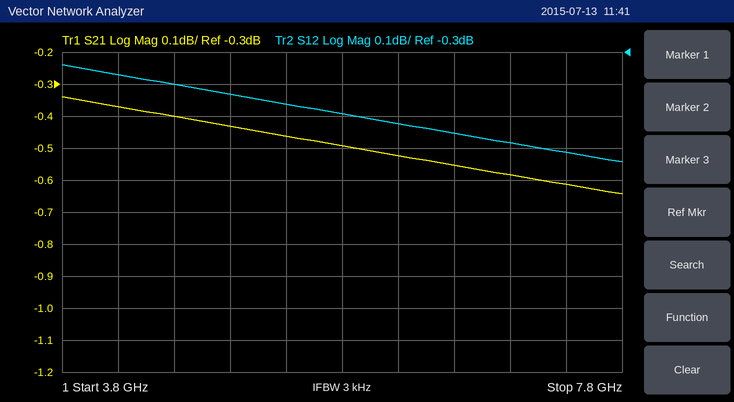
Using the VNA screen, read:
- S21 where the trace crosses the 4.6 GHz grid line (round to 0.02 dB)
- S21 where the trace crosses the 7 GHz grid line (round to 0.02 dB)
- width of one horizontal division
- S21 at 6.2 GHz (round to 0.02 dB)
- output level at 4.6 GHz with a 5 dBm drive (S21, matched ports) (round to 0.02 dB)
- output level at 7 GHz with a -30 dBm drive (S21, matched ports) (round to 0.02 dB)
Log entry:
-0.40 dB
-0.58 dB
400 MHz
-0.52 dB
4.60 dBm
-30.58 dBm
